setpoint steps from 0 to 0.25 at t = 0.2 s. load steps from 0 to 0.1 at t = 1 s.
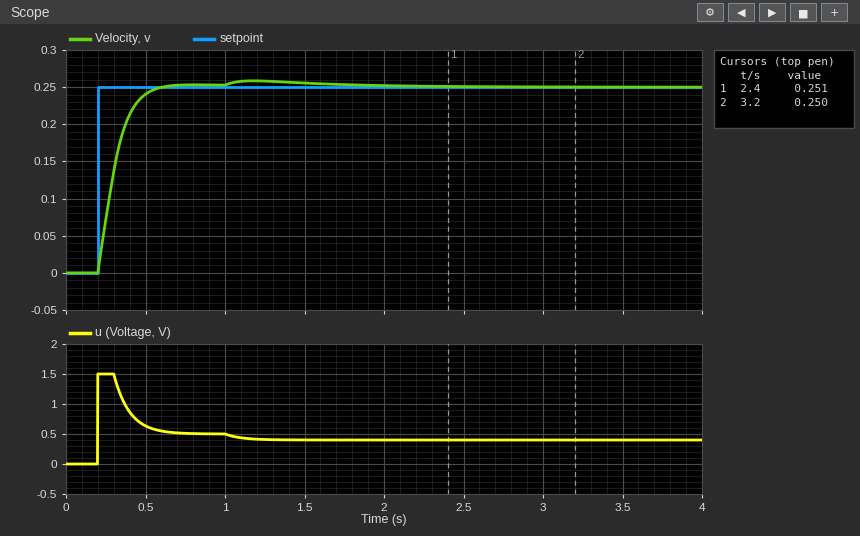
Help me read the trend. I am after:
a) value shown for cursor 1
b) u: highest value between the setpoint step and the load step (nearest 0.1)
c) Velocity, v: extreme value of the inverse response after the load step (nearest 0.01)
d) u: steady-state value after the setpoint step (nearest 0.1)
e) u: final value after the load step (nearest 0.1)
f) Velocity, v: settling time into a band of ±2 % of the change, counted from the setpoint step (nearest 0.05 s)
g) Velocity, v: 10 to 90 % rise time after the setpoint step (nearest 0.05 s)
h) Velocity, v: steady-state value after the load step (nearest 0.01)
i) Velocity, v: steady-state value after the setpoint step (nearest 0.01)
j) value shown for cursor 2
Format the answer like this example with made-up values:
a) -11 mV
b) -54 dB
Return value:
a) 0.251
b) 1.5
c) 0.26
d) 0.5
e) 0.4
f) 0.35 s
g) 0.20 s
h) 0.25
i) 0.25
j) 0.250
